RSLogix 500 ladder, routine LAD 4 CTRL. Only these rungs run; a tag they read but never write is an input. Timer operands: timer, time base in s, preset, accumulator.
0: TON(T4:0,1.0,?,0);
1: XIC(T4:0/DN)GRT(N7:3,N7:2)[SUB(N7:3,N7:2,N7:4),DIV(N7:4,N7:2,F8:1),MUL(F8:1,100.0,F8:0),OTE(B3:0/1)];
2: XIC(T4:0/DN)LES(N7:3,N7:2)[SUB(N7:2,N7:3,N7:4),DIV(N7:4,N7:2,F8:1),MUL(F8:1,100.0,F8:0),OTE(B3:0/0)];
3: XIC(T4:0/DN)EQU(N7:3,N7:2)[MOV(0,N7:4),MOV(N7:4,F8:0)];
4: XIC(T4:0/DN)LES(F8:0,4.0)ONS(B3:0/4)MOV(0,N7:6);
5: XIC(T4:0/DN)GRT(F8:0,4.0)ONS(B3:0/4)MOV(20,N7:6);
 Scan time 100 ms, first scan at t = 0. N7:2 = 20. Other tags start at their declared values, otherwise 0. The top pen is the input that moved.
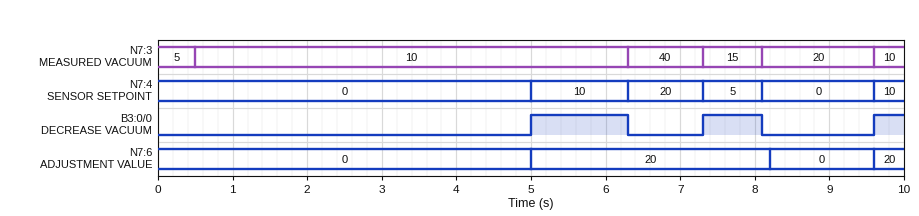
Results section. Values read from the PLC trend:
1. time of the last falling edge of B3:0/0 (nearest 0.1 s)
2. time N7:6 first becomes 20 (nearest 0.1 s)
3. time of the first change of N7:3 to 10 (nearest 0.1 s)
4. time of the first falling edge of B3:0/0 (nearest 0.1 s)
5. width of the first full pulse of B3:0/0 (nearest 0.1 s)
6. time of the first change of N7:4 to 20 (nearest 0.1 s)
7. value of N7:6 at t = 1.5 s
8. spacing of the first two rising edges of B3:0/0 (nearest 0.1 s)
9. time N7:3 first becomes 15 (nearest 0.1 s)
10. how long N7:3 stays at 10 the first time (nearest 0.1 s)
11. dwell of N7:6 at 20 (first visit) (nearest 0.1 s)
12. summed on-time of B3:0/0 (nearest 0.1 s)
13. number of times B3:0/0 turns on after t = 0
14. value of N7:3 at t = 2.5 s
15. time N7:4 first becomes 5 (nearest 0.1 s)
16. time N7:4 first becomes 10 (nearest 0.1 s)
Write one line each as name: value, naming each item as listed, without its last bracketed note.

time of the last falling edge of B3:0/0: 8.1 s
time N7:6 first becomes 20: 5.0 s
time of the first change of N7:3 to 10: 0.5 s
time of the first falling edge of B3:0/0: 6.3 s
width of the first full pulse of B3:0/0: 1.3 s
time of the first change of N7:4 to 20: 6.3 s
value of N7:6 at t = 1.5 s: 0
spacing of the first two rising edges of B3:0/0: 2.3 s
time N7:3 first becomes 15: 7.3 s
how long N7:3 stays at 10 the first time: 5.8 s
dwell of N7:6 at 20 (first visit): 3.2 s
summed on-time of B3:0/0: 2.5 s
number of times B3:0/0 turns on after t = 0: 3
value of N7:3 at t = 2.5 s: 10
time N7:4 first becomes 5: 7.3 s
time N7:4 first becomes 10: 5.0 s
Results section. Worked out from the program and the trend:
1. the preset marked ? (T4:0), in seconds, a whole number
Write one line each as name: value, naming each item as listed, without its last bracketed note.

the preset marked ? (T4:0), in seconds, a whole number: 5 s
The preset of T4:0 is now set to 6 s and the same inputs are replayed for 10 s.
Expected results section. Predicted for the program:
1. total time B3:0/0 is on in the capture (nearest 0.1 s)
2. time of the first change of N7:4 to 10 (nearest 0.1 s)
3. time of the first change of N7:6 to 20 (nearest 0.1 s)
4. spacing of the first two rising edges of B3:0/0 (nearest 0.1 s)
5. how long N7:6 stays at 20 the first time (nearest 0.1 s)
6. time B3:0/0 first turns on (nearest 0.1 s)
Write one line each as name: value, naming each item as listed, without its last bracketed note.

total time B3:0/0 is on in the capture: 1.5 s
time of the first change of N7:4 to 10: 6.0 s
time of the first change of N7:6 to 20: 6.0 s
spacing of the first two rising edges of B3:0/0: 1.3 s
how long N7:6 stays at 20 the first time: 2.2 s
time B3:0/0 first turns on: 6.0 s
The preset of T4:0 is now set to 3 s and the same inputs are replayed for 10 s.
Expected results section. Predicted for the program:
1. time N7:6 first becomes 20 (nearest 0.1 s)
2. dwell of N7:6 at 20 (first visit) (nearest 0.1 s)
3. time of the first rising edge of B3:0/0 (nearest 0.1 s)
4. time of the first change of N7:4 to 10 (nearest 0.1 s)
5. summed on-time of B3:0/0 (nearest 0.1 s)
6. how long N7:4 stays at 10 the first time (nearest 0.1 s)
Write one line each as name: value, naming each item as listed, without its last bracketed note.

time N7:6 first becomes 20: 3.0 s
dwell of N7:6 at 20 (first visit): 5.2 s
time of the first rising edge of B3:0/0: 3.0 s
time of the first change of N7:4 to 10: 3.0 s
summed on-time of B3:0/0: 4.5 s
how long N7:4 stays at 10 the first time: 3.3 s
